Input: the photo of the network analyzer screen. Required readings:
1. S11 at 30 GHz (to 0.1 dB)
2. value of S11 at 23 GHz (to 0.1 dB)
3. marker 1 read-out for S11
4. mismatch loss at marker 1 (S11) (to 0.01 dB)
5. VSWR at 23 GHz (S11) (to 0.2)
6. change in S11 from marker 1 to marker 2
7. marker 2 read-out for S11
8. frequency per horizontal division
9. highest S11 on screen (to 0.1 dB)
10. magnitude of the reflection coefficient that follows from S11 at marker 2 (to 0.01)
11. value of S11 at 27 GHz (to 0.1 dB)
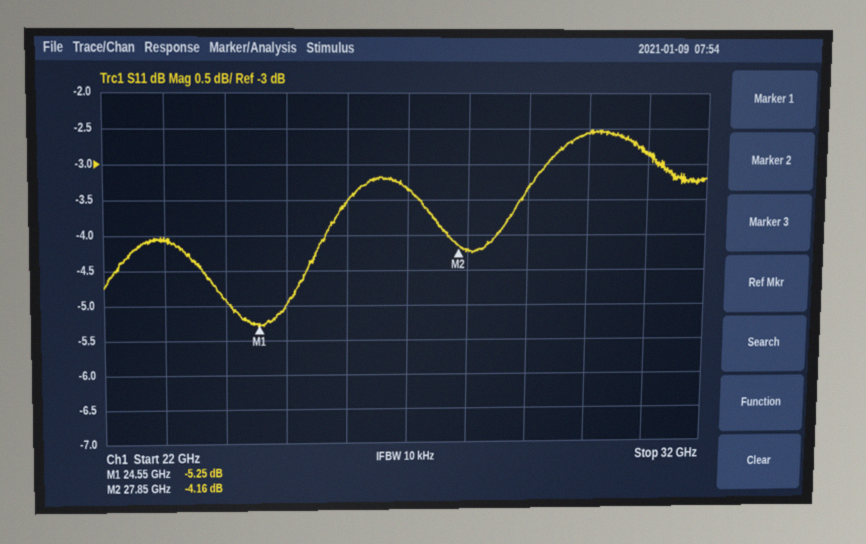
-2.6 dB
-4.1 dB
-5.25 dB
1.54 dB
4.4
1.09 dB
-4.16 dB
1 GHz
-2.5 dB
0.62
-3.3 dB
